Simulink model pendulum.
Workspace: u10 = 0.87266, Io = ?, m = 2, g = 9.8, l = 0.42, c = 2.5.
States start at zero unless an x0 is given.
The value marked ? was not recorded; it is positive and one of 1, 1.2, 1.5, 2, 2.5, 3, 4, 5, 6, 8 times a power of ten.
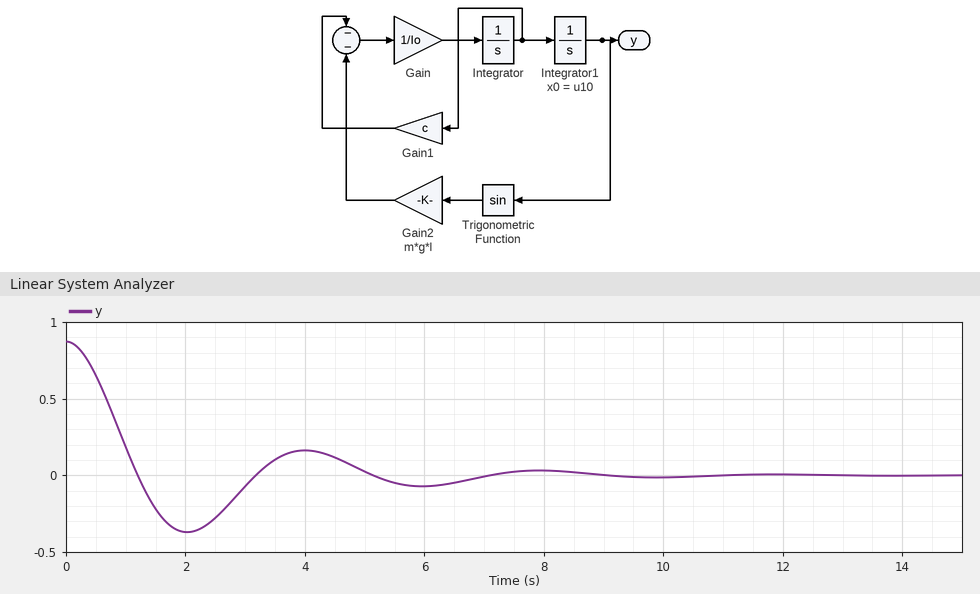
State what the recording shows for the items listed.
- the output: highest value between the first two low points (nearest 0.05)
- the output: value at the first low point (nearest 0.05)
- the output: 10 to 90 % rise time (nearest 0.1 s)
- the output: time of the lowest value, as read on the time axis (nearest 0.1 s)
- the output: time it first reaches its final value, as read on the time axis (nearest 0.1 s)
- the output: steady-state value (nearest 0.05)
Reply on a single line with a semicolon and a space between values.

0.15; -0.35; 0.8 s; 2.0 s; 1.2 s; 0.00
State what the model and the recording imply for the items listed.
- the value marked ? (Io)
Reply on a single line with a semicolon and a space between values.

3
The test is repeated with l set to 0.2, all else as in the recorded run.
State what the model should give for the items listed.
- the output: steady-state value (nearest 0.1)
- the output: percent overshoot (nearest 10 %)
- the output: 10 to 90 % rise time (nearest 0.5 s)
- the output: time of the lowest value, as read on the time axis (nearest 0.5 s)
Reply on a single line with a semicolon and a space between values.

0.0; 30 %; 1.5 s; 3.0 s
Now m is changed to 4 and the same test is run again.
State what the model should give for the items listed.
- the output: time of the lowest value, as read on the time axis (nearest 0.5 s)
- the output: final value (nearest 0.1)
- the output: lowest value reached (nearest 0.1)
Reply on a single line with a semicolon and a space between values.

1.5 s; 0.0; -0.5
